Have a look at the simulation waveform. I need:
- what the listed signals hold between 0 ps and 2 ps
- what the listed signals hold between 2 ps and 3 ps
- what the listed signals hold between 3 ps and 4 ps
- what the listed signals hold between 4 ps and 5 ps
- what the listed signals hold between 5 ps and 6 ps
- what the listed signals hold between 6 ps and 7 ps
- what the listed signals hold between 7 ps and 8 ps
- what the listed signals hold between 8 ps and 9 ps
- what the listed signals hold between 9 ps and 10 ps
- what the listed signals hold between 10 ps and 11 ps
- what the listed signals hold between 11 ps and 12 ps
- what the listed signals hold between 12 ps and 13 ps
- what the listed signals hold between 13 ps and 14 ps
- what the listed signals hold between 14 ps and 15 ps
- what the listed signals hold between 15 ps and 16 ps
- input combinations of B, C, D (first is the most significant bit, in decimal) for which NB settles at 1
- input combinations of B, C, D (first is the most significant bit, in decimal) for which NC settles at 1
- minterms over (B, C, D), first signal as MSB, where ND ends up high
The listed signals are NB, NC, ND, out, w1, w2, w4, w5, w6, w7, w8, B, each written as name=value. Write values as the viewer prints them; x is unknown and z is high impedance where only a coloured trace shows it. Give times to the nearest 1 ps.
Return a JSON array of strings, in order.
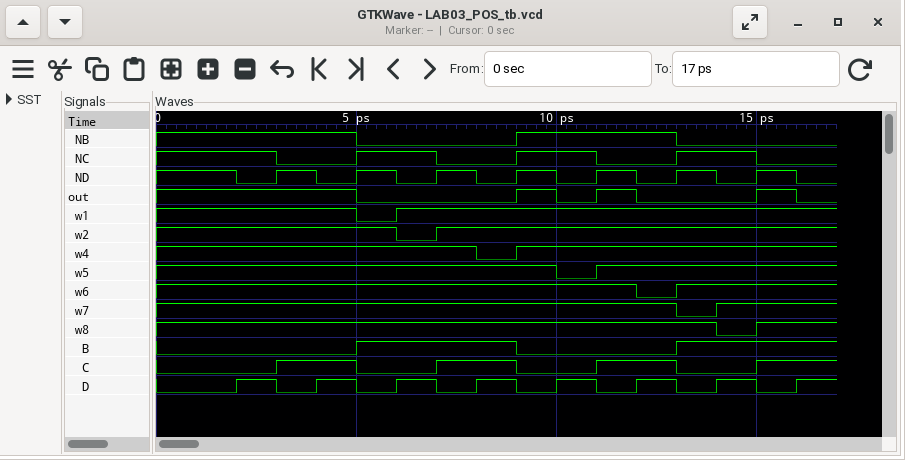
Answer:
["NB=1, NC=1, ND=1, out=1, w1=1, w2=1, w4=1, w5=1, w6=1, w7=1, w8=1, B=0", "NB=1, NC=1, ND=0, out=1, w1=1, w2=1, w4=1, w5=1, w6=1, w7=1, w8=1, B=0", "NB=1, NC=0, ND=1, out=1, w1=1, w2=1, w4=1, w5=1, w6=1, w7=1, w8=1, B=0", "NB=1, NC=0, ND=0, out=1, w1=1, w2=1, w4=1, w5=1, w6=1, w7=1, w8=1, B=0", "NB=0, NC=1, ND=1, out=0, w1=0, w2=1, w4=1, w5=1, w6=1, w7=1, w8=1, B=1", "NB=0, NC=1, ND=0, out=0, w1=1, w2=0, w4=1, w5=1, w6=1, w7=1, w8=1, B=1", "NB=0, NC=0, ND=1, out=0, w1=1, w2=1, w4=1, w5=1, w6=1, w7=1, w8=1, B=1", "NB=0, NC=0, ND=0, out=0, w1=1, w2=1, w4=0, w5=1, w6=1, w7=1, w8=1, B=1", "NB=1, NC=1, ND=1, out=1, w1=1, w2=1, w4=1, w5=1, w6=1, w7=1, w8=1, B=0", "NB=1, NC=1, ND=0, out=0, w1=1, w2=1, w4=1, w5=0, w6=1, w7=1, w8=1, B=0", "NB=1, NC=0, ND=1, out=1, w1=1, w2=1, w4=1, w5=1, w6=1, w7=1, w8=1, B=0", "NB=1, NC=0, ND=0, out=0, w1=1, w2=1, w4=1, w5=1, w6=0, w7=1, w8=1, B=0", "NB=0, NC=1, ND=1, out=0, w1=1, w2=1, w4=1, w5=1, w6=1, w7=0, w8=1, B=1", "NB=0, NC=1, ND=0, out=0, w1=1, w2=1, w4=1, w5=1, w6=1, w7=1, w8=0, B=1", "NB=0, NC=0, ND=1, out=1, w1=1, w2=1, w4=1, w5=1, w6=1, w7=1, w8=1, B=1", "0, 1, 2, 3", "0, 1, 4, 5", "0, 2, 4, 6"]
